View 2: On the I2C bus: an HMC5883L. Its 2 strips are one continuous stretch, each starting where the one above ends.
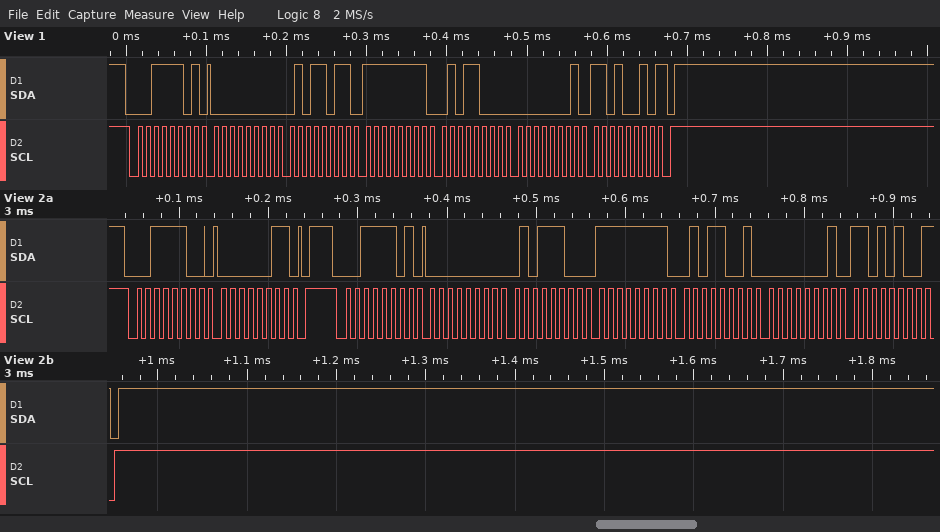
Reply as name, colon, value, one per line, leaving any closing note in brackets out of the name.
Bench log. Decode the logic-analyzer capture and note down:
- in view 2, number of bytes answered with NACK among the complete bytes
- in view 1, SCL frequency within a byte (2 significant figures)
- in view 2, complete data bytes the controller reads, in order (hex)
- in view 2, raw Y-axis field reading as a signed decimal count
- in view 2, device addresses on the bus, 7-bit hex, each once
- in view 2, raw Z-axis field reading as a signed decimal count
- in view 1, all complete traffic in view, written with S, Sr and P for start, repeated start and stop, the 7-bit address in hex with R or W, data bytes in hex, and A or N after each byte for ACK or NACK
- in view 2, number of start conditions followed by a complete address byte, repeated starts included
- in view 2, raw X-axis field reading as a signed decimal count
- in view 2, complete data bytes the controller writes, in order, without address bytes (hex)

in view 2, number of bytes answered with NACK among the complete bytes: 1
in view 1, SCL frequency within a byte: 100 kHz
in view 2, complete data bytes the controller reads, in order: 00 5C FF 59 01 D4
in view 2, raw Y-axis field reading as a signed decimal count: 468
in view 2, device addresses on the bus, 7-bit hex, each once: 0x1E
in view 2, raw Z-axis field reading as a signed decimal count: -167
in view 1, all complete traffic in view, written with S, Sr and P for start, repeated start and stop, the 7-bit address in hex with R or W, data bytes in hex, and A or N after each byte for ACK or NACK: S 1ER A 00 A 5B A FF A 58 A 01 A D2 N P
in view 2, number of start conditions followed by a complete address byte, repeated starts included: 2
in view 2, raw X-axis field reading as a signed decimal count: 92
in view 2, complete data bytes the controller writes, in order, without address bytes: 03
